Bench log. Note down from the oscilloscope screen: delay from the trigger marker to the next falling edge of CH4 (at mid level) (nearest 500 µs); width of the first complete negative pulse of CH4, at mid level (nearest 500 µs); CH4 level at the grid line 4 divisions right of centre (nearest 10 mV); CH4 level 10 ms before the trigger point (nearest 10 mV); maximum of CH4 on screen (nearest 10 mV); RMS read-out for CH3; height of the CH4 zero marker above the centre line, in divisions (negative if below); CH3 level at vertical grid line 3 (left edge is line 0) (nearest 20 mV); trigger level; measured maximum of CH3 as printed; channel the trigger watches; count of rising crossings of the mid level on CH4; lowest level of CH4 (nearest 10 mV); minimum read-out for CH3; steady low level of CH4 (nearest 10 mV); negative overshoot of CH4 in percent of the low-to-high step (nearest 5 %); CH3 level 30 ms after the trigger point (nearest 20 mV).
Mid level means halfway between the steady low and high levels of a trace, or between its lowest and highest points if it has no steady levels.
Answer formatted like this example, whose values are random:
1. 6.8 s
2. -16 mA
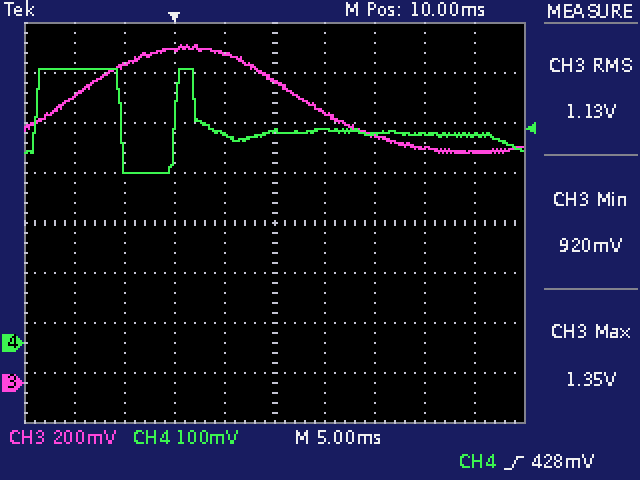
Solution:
1. 2.0 ms
2. 5.5 ms
3. 420 mV
4. 550 mV
5. 550 mV
6. 1.13 V
7. -2.4 div
8. 1.34 V
9. 428 mV
10. 1.35 V
11. CH4
12. 2
13. 340 mV
14. 920 mV
15. 420 mV
16. 60 %
17. 920 mV
